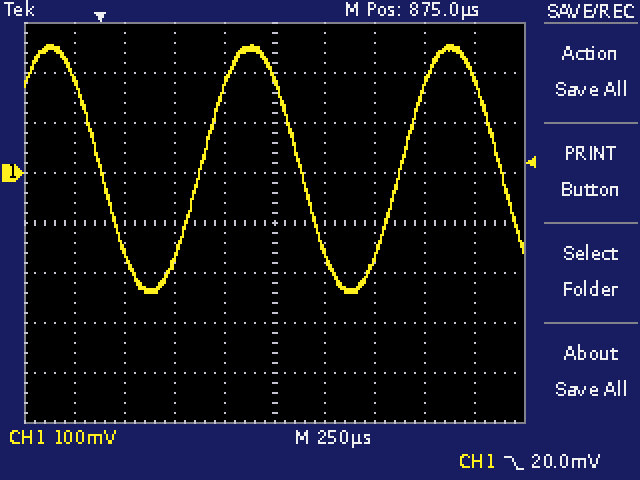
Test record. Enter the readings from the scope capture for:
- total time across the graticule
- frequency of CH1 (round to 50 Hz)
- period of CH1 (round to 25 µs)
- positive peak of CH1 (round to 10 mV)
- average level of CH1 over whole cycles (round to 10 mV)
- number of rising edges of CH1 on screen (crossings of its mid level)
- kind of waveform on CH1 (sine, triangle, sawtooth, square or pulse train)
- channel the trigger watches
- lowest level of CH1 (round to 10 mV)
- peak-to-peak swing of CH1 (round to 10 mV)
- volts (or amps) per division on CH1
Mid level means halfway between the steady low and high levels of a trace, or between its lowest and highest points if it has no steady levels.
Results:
2.5 ms
1.00 kHz
1.000 ms
260 mV
10 mV
2
sine
CH1
-240 mV
500 mV
100 mV
